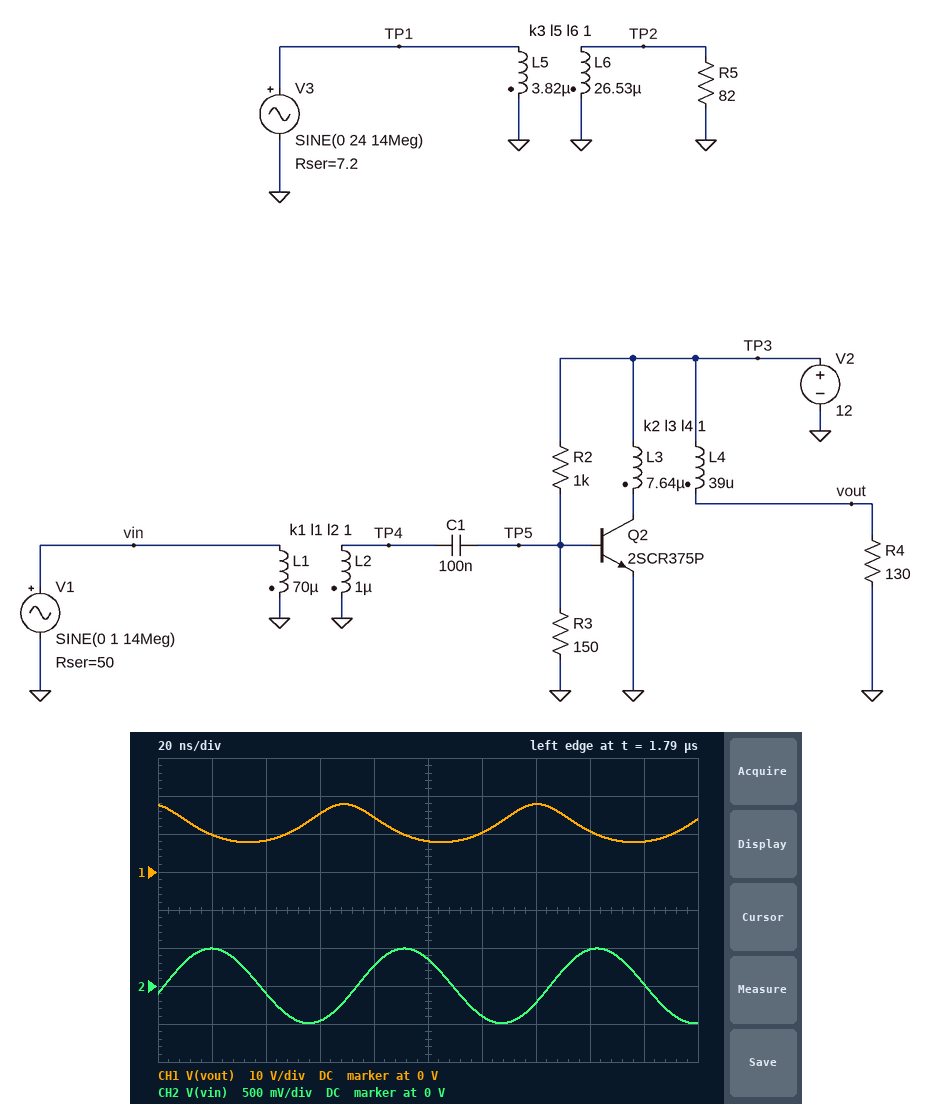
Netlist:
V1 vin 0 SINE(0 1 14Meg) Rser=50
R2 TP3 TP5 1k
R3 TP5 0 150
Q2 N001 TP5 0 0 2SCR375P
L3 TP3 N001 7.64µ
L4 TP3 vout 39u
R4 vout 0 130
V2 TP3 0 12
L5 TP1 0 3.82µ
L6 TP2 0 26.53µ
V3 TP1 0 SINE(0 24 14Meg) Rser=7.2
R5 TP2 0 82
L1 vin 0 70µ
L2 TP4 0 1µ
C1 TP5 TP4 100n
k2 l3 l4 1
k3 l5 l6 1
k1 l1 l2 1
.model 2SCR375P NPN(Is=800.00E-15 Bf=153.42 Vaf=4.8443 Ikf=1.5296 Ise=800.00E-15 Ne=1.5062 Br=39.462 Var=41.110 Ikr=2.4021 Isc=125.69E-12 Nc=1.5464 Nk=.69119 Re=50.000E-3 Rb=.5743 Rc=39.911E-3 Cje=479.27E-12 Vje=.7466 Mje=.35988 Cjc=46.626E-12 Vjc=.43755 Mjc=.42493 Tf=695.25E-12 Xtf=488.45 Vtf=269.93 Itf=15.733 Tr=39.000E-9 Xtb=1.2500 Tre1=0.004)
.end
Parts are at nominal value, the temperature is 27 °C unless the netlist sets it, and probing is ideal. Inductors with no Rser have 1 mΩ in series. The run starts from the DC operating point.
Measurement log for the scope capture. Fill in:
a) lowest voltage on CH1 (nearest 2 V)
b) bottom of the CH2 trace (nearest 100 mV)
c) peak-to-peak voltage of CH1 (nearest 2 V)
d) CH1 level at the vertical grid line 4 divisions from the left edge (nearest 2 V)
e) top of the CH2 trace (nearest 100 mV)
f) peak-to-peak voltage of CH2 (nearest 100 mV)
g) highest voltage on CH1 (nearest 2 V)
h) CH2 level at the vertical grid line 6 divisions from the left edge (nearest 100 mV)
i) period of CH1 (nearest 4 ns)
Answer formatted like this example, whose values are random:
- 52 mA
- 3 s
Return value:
- 8 V
- -500 mV
- 10 V
- 14 V
- 500 mV
- 1.0 V
- 18 V
- -400 mV
- 72 ns
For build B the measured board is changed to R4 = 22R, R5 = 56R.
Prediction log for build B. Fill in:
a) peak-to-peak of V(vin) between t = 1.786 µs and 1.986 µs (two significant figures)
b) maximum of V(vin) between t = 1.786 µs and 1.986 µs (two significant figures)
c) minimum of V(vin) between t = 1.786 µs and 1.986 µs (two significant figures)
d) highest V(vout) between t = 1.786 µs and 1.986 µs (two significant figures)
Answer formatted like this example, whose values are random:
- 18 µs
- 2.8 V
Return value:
- 1.0 V
- 500 mV
- -500 mV
- 14 V
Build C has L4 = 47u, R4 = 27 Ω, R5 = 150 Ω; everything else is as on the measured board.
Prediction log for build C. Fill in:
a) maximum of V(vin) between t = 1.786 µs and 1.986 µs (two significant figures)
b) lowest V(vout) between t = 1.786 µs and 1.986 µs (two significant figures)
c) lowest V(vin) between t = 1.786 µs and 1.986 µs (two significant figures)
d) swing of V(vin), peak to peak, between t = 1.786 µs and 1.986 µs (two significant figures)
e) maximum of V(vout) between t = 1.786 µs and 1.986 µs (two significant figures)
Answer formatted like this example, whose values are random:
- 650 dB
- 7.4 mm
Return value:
- 500 mV
- 10 V
- -500 mV
- 1.0 V
- 14 V
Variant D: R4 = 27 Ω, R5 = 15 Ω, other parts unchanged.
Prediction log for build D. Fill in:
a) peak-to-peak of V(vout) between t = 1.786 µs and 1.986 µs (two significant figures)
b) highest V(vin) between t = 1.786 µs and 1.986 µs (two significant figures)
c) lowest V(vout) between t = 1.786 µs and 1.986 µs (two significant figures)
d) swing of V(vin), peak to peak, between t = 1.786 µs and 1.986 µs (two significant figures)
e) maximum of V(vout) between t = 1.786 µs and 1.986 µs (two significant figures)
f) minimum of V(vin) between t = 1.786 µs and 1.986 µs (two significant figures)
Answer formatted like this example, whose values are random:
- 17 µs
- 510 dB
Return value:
- 4.1 V
- 500 mV
- 10 V
- 1.0 V
- 14 V
- -500 mV
